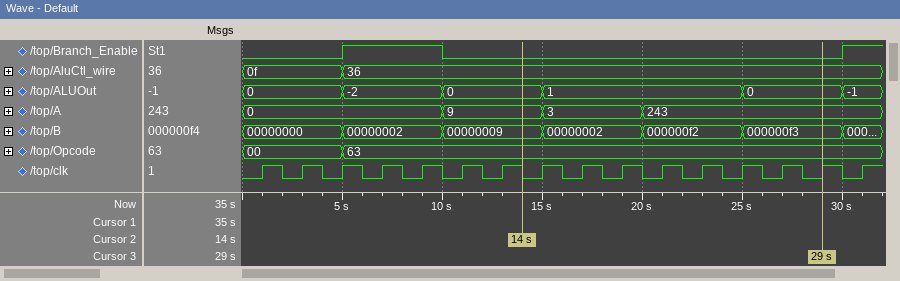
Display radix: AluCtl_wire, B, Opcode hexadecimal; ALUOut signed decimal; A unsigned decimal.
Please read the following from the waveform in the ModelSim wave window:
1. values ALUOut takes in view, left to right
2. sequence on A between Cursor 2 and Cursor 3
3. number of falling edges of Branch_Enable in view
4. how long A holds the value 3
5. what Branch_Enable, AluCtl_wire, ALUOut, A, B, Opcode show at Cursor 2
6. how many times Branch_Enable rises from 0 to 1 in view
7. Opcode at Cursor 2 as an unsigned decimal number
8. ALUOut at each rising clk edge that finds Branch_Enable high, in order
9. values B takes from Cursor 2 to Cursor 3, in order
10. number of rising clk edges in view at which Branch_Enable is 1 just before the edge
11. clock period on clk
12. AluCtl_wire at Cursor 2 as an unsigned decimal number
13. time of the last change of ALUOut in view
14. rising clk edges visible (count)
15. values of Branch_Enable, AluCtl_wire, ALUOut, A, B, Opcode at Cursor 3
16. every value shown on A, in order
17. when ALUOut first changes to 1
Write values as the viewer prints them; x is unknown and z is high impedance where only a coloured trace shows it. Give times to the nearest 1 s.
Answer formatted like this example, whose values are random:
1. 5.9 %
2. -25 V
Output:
1. 0, -2, 0, 1, 0, -1
2. 9, 3, 243
3. 1
4. 5 s
5. Branch_Enable=0, AluCtl_wire=36, ALUOut=0, A=9, B=00000009, Opcode=63
6. 2
7. 99
8. -2, -2, -1
9. 00000009, 00000002, 000000f2, 000000f3
10. 3
11. 2 s
12. 54
13. 30 s
14. 16
15. Branch_Enable=0, AluCtl_wire=36, ALUOut=0, A=243, B=000000f3, Opcode=63
16. 0, 9, 3, 243
17. 15 s
